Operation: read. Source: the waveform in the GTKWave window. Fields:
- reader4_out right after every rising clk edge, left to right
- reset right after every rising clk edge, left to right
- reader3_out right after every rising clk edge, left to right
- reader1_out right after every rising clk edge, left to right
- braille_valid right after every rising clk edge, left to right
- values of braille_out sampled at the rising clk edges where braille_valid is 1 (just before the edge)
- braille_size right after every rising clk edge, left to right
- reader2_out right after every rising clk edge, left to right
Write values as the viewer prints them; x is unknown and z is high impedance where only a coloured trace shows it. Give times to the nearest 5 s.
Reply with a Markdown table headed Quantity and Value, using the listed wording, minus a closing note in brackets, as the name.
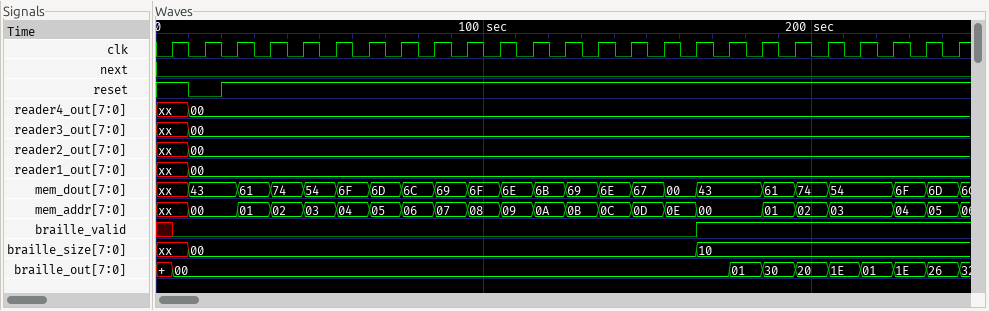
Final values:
| Quantity | Value |
|---|---|
| reader4_out right after every rising clk edge, left to right | xx, 00, 00, 00, 00, 00, 00, 00, 00, 00, 00, 00, 00, 00, 00, 00, 00, 00, 00, 00, 00, 00, 00, 00, 00 |
| reset right after every rising clk edge, left to right | 1 0 1 1 1 1 1 1 1 1 1 1 1 1 1 1 1 1 1 1 1 1 1 1 1 |
| reader3_out right after every rising clk edge, left to right | xx, 00, 00, 00, 00, 00, 00, 00, 00, 00, 00, 00, 00, 00, 00, 00, 00, 00, 00, 00, 00, 00, 00, 00, 00 |
| reader1_out right after every rising clk edge, left to right | xx, 00, 00, 00, 00, 00, 00, 00, 00, 00, 00, 00, 00, 00, 00, 00, 00, 00, 00, 00, 00, 00, 00, 00, 00 |
| braille_valid right after every rising clk edge, left to right | 0 0 0 0 0 0 0 0 0 0 0 0 0 0 0 0 1 1 1 1 1 1 1 1 1 |
| values of braille_out sampled at the rising clk edges where braille_valid is 1 | 00, 01, 30, 20, 1E, 01, 1E, 26 |
| braille_size right after every rising clk edge, left to right | xx, 00, 00, 00, 00, 00, 00, 00, 00, 00, 00, 00, 00, 00, 00, 00, 10, 10, 10, 10, 10, 10, 10, 10, 10 |
| reader2_out right after every rising clk edge, left to right | xx, 00, 00, 00, 00, 00, 00, 00, 00, 00, 00, 00, 00, 00, 00, 00, 00, 00, 00, 00, 00, 00, 00, 00, 00 |
